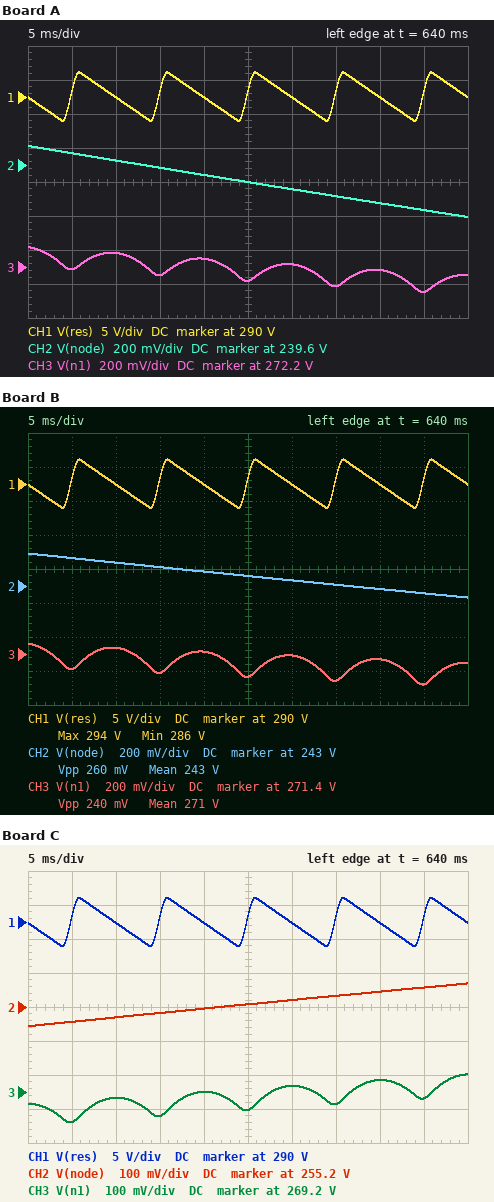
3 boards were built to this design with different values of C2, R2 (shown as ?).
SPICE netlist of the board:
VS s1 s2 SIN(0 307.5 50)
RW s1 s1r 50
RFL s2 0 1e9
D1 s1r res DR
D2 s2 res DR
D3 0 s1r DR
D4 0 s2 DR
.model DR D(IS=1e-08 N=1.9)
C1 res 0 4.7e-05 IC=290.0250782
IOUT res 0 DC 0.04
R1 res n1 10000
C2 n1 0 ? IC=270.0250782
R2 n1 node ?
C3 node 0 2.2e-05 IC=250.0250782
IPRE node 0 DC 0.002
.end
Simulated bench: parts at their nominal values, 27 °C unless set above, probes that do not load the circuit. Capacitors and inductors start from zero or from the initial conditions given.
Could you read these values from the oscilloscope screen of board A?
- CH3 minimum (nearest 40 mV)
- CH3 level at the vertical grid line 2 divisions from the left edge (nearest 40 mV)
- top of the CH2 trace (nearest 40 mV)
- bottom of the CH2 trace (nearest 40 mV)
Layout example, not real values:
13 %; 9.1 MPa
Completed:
272.04 V; 272.28 V; 239.72 V; 239.28 V
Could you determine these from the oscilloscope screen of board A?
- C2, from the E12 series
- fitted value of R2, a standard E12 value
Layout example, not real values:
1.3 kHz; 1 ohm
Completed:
8.2 µF; 18 kΩ
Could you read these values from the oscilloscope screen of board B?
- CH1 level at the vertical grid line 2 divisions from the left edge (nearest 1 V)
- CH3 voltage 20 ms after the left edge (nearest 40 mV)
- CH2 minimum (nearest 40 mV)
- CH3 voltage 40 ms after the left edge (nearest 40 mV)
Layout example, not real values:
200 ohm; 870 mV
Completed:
290 V; 271.40 V; 242.92 V; 271.36 V
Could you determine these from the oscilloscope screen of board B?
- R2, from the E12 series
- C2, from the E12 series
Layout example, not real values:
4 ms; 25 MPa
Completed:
15 kΩ; 6.8 µF
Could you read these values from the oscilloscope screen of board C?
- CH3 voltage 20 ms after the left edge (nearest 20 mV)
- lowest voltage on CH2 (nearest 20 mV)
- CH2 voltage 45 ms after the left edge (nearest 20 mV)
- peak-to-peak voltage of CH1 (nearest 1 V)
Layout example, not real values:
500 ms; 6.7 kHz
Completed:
269.20 V; 255.14 V; 255.26 V; 7 V
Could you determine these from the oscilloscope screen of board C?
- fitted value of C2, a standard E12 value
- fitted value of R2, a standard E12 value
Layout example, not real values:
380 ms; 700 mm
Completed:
15 µF; 6.8 kΩ
